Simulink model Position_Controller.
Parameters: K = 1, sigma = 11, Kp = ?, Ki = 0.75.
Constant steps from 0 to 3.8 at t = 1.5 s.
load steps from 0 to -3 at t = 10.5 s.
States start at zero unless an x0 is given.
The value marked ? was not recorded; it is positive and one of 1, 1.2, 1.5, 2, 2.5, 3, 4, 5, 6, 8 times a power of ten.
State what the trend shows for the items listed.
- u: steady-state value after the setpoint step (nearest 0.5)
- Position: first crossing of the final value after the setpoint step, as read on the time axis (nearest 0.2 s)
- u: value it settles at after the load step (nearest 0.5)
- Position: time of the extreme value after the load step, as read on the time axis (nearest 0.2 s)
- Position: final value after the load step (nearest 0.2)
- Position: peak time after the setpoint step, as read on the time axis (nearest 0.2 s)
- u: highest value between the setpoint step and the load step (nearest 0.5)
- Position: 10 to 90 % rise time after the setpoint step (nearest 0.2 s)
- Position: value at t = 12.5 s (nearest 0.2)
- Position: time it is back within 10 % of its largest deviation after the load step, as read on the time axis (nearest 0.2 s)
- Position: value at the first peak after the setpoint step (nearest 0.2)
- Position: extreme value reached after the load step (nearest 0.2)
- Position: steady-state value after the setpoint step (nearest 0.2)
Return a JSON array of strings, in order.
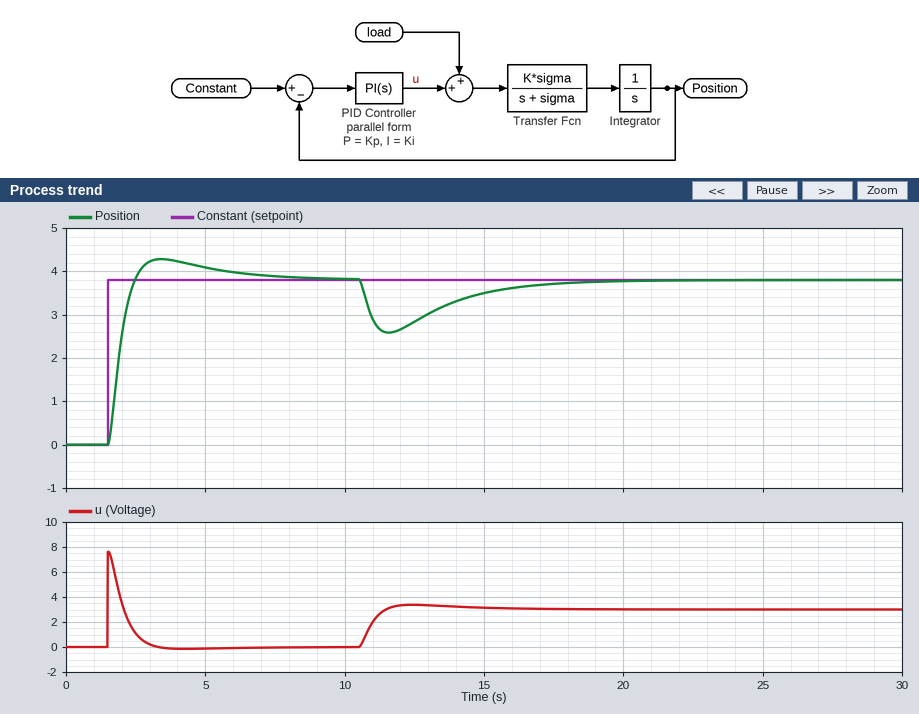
["0.0", "2.4 s", "3.0", "11.6 s", "3.8", "3.4 s", "7.5", "0.6 s", "2.8", "16.8 s", "4.2", "2.6", "3.8"]
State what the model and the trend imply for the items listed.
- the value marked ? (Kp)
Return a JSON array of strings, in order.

["2"]
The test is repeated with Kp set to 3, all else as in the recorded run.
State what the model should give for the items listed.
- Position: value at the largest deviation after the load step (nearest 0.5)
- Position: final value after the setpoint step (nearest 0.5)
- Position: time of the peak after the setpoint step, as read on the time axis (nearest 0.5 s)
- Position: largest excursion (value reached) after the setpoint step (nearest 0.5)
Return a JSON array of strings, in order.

["3.0", "4.0", "3.0 s", "4.0"]
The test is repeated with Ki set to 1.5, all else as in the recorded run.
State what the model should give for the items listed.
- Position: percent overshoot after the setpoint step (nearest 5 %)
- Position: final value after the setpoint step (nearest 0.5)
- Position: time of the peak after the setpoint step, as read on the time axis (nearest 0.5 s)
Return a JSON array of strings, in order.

["20 %", "4.0", "3.0 s"]
